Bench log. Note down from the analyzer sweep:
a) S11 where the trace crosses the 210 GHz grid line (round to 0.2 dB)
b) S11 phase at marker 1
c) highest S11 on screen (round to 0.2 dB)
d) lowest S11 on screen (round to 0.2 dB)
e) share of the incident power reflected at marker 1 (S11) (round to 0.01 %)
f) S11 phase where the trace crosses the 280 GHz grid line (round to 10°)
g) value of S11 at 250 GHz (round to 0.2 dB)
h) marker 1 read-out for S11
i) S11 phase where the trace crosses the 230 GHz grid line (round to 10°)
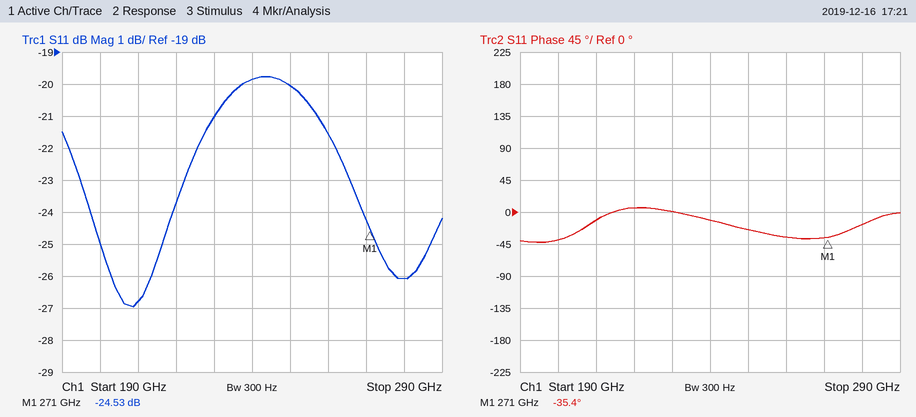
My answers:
-26.8 dB
-35.4°
-19.8 dB
-27.0 dB
0.35 %
-20°
-20.0 dB
-24.53 dB
0°
